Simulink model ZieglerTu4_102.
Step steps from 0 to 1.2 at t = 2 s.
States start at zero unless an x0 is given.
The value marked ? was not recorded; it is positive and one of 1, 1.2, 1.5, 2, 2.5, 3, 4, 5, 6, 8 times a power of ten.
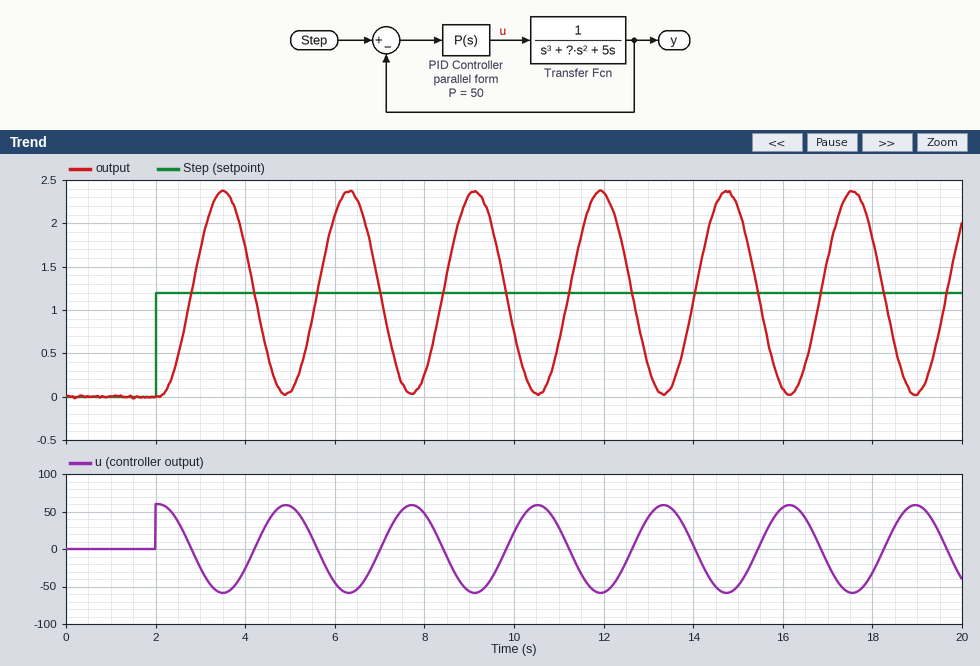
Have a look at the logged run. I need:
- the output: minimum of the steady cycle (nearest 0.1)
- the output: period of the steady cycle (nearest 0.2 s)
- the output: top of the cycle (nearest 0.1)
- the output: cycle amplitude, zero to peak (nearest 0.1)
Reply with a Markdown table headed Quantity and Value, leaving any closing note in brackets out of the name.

| Quantity | Value |
|---|---|
| the output: minimum of the steady cycle | 0.0 |
| the output: period of the steady cycle | 2.8 s |
| the output: top of the cycle | 2.4 |
| the output: cycle amplitude, zero to peak | 1.2 |
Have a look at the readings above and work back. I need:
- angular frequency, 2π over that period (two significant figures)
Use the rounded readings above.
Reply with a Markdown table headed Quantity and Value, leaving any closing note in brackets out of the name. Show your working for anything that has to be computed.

| Quantity | Value |
|---|---|
| angular frequency, 2π over that period | 2π / 2.8 = 2.2 rad/s |
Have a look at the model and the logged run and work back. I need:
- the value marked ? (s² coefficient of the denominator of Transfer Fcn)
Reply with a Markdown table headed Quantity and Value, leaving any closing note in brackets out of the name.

| Quantity | Value |
|---|---|
| the value marked ? | 10 |
